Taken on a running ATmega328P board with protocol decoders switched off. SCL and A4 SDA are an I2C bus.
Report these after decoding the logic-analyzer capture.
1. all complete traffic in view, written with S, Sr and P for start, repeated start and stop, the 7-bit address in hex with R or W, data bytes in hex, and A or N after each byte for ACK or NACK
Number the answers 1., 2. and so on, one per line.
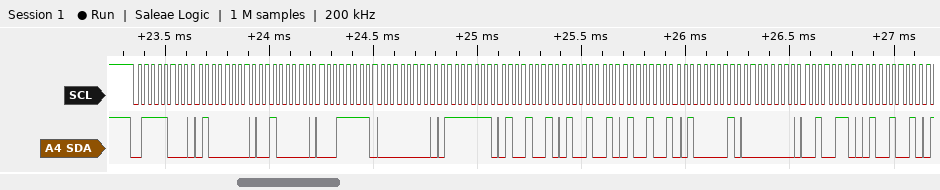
1. S 3CW A 40 A 20 A 1F A 00 A 7F A 49 A 49 A 49 A 41 A 00 A 26 A 49 A
